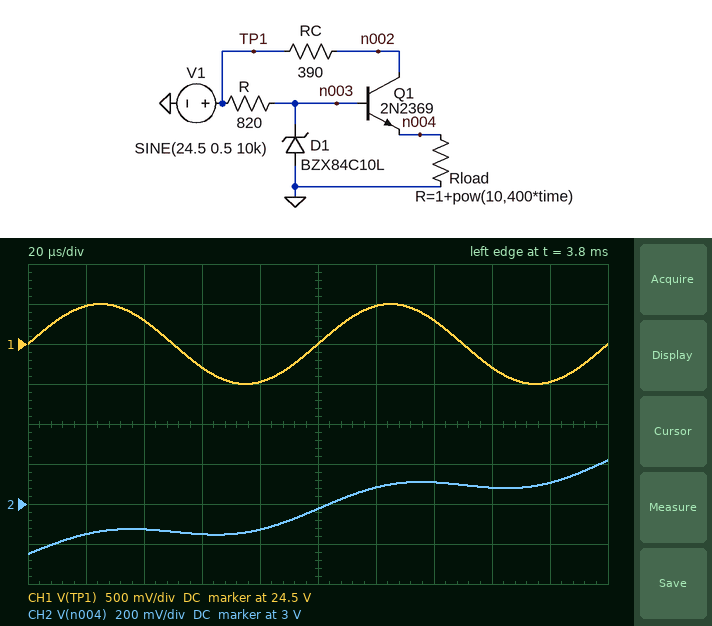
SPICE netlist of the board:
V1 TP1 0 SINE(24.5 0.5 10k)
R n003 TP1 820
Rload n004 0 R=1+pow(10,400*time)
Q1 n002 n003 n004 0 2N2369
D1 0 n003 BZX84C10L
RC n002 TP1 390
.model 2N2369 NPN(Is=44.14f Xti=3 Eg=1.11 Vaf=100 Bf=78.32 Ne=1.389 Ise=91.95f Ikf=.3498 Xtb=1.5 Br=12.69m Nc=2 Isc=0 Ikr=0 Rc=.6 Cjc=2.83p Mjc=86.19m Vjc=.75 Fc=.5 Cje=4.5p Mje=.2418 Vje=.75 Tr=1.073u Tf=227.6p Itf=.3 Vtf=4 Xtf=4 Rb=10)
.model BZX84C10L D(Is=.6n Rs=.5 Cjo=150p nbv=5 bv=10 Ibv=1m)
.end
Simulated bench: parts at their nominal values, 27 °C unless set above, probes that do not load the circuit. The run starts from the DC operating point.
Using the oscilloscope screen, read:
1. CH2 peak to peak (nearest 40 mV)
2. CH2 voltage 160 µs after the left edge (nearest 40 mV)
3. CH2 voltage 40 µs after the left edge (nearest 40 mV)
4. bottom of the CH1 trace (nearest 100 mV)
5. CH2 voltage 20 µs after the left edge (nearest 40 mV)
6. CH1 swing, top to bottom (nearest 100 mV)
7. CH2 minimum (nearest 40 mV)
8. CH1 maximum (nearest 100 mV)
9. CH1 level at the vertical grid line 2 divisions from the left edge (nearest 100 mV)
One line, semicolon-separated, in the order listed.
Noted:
480 mV; 3.08 V; 2.88 V; 24.0 V; 2.84 V; 1.0 V; 2.76 V; 25.0 V; 24.8 V
